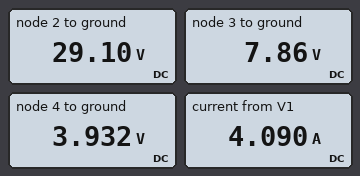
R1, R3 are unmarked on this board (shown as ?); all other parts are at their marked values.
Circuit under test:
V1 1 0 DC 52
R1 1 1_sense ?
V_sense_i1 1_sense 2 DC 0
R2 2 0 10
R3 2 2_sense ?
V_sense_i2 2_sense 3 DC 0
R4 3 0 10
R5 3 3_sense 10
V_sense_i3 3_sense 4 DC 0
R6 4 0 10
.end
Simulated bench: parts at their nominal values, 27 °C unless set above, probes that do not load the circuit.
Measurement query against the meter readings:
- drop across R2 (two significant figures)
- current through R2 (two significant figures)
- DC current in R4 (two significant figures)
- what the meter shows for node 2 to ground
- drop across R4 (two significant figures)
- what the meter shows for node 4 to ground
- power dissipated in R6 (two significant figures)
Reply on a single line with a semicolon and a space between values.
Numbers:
29 V; 2.9 A; 790 mA; 29.10 V; 7.9 V; 3.932 V; 1.5 W
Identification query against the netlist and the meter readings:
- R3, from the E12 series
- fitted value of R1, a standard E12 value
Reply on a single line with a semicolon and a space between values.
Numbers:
18 Ω; 5.6 Ω
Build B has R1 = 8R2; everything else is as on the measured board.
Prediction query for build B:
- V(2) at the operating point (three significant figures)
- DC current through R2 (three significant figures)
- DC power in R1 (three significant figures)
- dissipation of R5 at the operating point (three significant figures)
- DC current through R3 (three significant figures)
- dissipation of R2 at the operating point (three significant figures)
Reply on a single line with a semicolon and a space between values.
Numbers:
24.2 V; 2.42 A; 94.5 W; 1.07 W; 979 mA; 58.4 W
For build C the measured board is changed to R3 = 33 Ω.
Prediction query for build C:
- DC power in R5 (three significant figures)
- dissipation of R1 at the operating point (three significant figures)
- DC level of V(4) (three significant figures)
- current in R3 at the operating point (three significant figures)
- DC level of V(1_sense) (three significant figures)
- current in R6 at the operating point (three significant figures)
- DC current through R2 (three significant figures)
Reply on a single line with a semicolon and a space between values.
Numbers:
660 mW; 82.0 W; 2.57 V; 771 mA; 30.6 V; 257 mA; 3.06 A
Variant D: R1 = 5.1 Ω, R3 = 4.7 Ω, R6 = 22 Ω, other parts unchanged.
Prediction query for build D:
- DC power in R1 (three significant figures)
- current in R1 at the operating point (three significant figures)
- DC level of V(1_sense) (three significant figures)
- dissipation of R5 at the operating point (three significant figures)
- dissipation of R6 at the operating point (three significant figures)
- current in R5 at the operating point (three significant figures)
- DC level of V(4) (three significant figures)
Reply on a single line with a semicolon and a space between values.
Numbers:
122 W; 4.90 A; 27.0 V; 2.73 W; 6.00 W; 522 mA; 11.5 V
